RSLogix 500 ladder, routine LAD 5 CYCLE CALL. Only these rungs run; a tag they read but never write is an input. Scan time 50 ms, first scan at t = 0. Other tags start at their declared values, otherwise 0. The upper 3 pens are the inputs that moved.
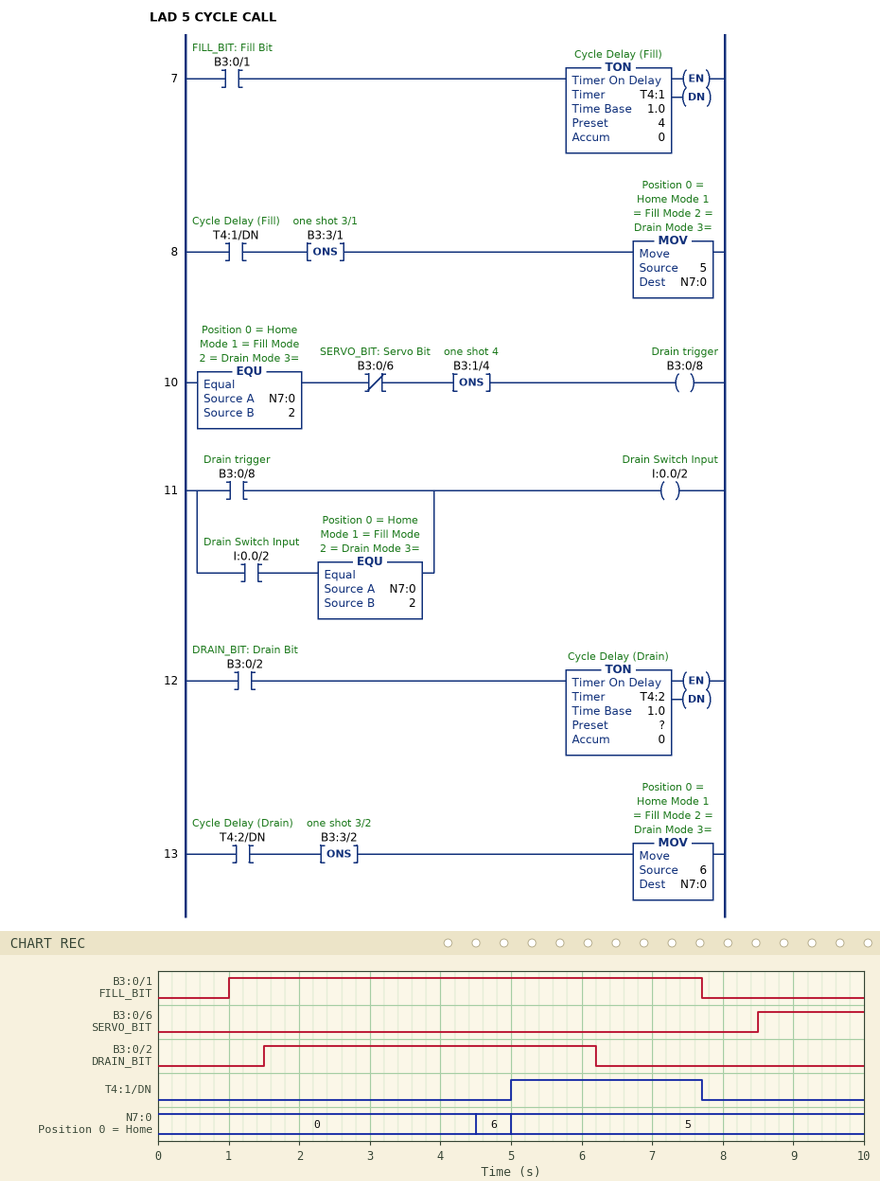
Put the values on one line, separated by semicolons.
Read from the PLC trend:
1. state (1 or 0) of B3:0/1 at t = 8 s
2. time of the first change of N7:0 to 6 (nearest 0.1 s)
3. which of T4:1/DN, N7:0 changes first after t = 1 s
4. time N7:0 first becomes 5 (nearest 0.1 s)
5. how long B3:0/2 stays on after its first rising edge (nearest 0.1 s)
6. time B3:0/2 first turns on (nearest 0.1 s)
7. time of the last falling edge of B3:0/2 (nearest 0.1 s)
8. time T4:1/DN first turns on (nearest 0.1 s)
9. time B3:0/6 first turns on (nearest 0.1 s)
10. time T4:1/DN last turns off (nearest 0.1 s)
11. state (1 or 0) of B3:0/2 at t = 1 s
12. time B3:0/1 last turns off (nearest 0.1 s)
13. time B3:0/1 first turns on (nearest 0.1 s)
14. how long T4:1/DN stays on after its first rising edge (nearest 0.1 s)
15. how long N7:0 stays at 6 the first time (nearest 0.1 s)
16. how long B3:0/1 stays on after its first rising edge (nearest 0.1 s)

0; 4.5 s; N7:0; 5.0 s; 4.7 s; 1.5 s; 6.2 s; 5.0 s; 8.5 s; 7.7 s; 0; 7.7 s; 1.0 s; 2.7 s; 0.5 s; 6.7 s
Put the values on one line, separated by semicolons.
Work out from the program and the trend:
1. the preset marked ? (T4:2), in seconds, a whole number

3 s
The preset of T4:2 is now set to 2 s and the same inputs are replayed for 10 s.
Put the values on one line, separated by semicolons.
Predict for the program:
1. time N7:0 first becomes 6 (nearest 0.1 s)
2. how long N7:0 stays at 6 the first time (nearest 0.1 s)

3.5 s; 1.5 s
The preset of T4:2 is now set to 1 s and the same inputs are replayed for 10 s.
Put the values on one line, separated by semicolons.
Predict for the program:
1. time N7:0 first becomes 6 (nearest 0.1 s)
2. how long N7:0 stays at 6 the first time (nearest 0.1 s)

2.5 s; 2.5 s
